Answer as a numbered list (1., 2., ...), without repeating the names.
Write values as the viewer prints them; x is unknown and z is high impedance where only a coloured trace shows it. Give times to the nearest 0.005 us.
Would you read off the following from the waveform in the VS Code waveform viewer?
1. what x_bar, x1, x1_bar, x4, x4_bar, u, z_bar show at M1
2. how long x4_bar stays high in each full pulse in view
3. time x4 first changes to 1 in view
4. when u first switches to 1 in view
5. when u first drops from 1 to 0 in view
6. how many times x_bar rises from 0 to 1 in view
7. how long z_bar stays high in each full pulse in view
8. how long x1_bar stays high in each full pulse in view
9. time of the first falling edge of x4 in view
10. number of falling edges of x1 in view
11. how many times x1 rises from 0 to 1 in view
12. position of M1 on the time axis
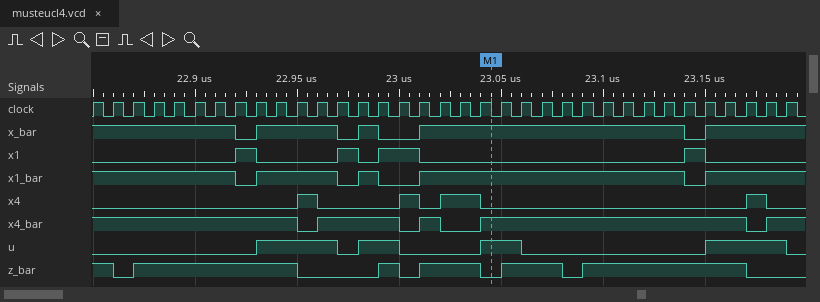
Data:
1. x_bar=1, x1=0, x1_bar=1, x4=0, x4_bar=1, u=1, z_bar=0
2. 0.04 us, 0.01 us, 0.13 us
3. 22.95 us
4. 22.93 us
5. 22.97 us
6. 4
7. 0.08 us, 0.01 us, 0.03 us, 0.03 us, 0.08 us
8. 0.04 us, 0.01 us, 0.13 us
9. 22.96 us
10. 4
11. 4
12. 23.045 us
